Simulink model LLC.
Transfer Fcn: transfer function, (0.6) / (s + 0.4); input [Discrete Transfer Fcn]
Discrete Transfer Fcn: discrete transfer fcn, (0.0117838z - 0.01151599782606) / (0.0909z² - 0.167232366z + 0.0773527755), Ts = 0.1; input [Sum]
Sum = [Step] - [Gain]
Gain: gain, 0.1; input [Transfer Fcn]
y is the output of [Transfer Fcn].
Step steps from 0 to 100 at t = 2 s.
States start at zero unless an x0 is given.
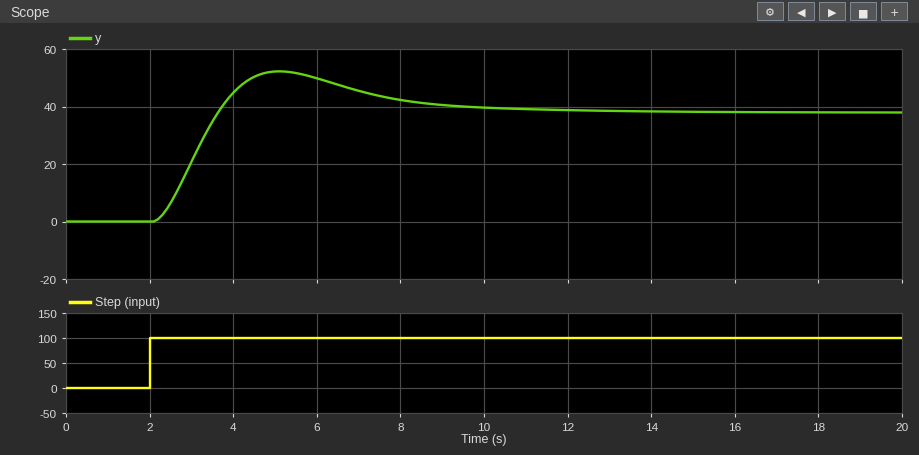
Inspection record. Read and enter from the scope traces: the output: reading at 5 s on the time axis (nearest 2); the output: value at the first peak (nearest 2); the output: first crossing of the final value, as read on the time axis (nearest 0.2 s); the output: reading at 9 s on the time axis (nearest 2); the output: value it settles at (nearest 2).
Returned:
52
52
3.6 s
40
38
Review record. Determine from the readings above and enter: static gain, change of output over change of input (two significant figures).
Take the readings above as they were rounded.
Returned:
0.38
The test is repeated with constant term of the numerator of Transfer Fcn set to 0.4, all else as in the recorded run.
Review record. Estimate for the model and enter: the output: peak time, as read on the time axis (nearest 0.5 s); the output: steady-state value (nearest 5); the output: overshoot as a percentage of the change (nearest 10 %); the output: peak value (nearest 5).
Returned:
5.0 s
25
40 %
35
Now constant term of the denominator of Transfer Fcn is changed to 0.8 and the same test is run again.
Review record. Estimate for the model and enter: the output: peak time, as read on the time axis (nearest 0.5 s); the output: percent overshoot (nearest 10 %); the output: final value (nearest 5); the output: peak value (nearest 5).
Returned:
4.5 s
80 %
20
35
